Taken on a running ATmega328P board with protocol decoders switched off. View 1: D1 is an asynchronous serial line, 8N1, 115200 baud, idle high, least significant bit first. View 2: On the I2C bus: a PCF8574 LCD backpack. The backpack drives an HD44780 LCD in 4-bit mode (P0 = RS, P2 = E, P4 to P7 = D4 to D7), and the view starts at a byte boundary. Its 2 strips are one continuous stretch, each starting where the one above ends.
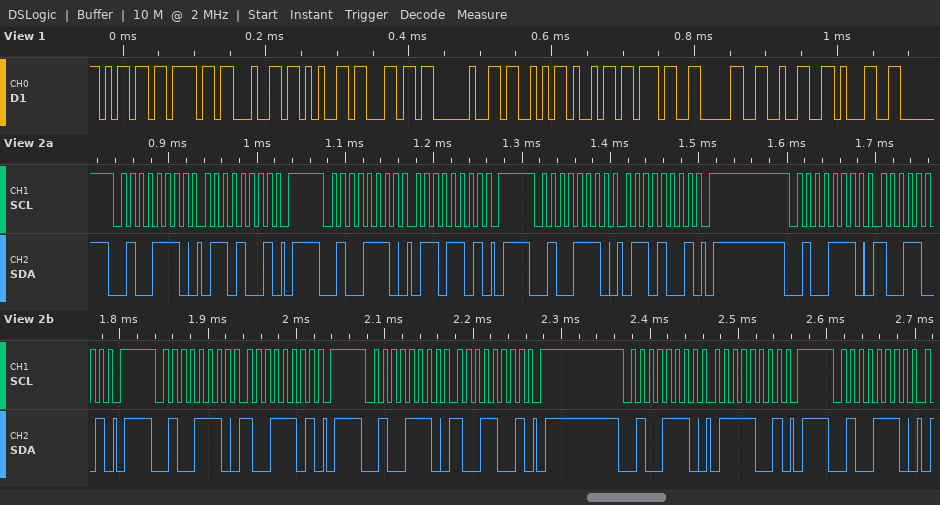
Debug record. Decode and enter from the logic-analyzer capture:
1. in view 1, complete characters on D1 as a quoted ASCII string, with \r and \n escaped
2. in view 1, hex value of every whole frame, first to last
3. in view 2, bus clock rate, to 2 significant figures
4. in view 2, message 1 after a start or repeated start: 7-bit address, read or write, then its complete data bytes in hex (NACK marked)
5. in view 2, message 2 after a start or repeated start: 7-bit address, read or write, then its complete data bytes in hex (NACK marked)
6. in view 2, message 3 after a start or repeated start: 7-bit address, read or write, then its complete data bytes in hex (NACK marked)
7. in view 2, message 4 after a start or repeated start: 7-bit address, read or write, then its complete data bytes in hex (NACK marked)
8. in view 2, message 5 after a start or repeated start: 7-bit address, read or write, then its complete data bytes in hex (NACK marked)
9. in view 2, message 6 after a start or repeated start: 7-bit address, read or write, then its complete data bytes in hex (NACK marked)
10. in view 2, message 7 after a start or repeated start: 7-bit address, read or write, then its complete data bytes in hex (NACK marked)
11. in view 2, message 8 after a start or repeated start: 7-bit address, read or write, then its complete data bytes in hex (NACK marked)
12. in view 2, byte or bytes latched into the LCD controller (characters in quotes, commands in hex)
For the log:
"model Si7021"
0x6D 0x6F 0x64 0x65 0x6C 0x20 0x53 0x69 0x37 0x30 0x32 0x31
100 kHz
0x27 write: 69
0x27 write: 6D
0x27 write: 69
0x27 write: 99
0x27 write: 9D
0x27 write: 99
0x27 write: 79
0x27 write
'i'
